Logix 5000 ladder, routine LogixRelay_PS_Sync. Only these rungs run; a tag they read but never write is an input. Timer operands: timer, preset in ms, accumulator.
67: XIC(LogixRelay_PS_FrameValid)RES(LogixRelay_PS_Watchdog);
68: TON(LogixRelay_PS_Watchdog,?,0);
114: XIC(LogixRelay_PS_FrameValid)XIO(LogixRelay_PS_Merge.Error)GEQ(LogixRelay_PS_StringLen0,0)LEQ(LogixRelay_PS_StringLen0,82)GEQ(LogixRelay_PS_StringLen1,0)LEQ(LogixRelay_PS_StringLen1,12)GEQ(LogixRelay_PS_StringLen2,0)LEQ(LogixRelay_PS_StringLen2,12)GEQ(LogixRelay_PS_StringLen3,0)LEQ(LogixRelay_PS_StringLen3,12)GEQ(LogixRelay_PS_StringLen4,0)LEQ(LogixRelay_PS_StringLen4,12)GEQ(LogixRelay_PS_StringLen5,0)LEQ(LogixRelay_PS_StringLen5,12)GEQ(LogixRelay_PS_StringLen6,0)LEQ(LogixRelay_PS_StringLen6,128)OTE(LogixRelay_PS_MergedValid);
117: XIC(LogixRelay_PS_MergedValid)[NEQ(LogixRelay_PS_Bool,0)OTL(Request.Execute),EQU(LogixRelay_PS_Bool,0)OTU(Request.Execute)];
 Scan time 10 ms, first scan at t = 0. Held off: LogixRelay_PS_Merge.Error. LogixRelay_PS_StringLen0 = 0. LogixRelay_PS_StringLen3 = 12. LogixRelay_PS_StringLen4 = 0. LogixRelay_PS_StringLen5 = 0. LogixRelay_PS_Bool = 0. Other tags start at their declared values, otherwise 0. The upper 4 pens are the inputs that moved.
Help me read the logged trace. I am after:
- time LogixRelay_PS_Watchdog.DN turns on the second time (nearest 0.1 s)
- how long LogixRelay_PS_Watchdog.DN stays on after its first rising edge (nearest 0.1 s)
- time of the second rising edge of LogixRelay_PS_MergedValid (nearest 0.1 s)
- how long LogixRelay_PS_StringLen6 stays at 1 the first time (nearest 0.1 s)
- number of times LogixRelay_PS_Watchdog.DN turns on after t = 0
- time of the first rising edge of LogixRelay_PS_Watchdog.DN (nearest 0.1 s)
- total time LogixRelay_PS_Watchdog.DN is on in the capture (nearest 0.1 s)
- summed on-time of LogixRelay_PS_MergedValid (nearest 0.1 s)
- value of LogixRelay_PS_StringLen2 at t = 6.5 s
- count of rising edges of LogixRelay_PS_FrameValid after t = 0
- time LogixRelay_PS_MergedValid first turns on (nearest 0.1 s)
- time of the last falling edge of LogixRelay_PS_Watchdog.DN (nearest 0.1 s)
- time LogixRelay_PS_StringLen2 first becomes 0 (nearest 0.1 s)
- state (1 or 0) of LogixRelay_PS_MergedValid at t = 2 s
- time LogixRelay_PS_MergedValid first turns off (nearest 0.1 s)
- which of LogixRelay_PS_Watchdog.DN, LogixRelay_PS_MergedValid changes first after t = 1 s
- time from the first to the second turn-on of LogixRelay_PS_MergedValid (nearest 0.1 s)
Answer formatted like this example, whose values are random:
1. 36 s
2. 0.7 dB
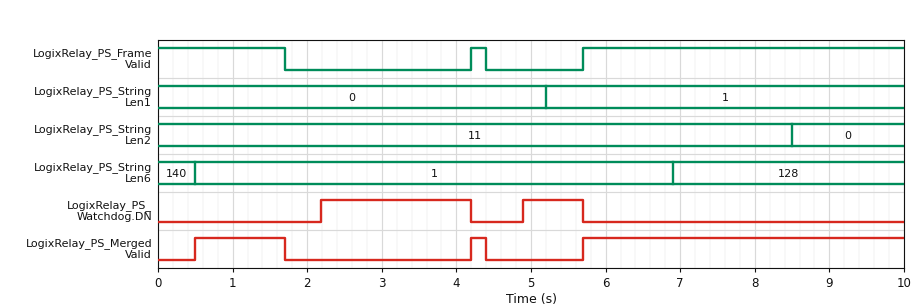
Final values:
1. 4.9 s
2. 2.0 s
3. 4.2 s
4. 6.4 s
5. 2
6. 2.2 s
7. 2.8 s
8. 5.7 s
9. 11
10. 2
11. 0.5 s
12. 5.7 s
13. 8.5 s
14. 0
15. 1.7 s
16. LogixRelay_PS_MergedValid
17. 3.7 s
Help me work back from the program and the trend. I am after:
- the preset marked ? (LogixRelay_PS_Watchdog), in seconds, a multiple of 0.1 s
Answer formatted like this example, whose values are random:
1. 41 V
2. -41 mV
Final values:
1. 0.5 s
